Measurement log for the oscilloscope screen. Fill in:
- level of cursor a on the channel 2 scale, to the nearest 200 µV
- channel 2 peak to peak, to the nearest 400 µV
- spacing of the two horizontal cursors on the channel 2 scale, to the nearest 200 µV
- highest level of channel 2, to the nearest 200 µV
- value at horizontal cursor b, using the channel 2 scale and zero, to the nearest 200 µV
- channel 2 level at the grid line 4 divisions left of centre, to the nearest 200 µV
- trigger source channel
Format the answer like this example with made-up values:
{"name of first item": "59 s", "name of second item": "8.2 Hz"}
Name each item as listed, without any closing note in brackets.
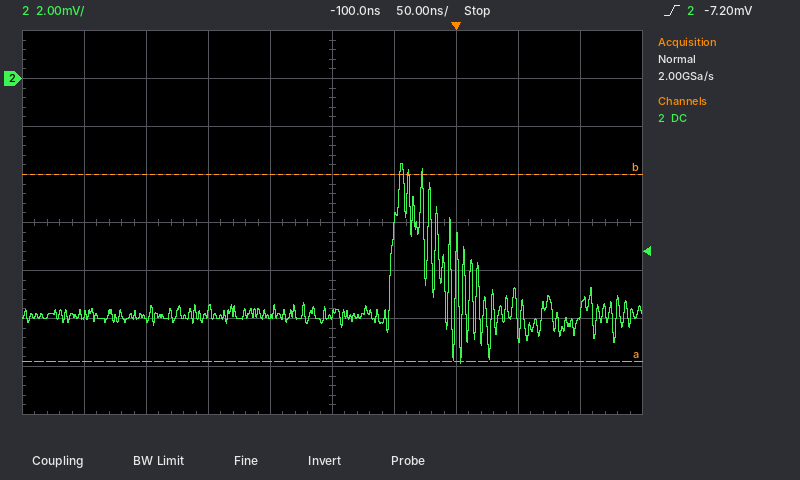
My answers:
{"level of cursor a on the channel 2 scale, to the nearest 200 µV": "-11.8 mV", "channel 2 peak to peak, to the nearest 400 µV": "8.4 mV", "spacing of the two horizontal cursors on the channel 2 scale, to the nearest 200 µV": "7.8 mV", "highest level of channel 2, to the nearest 200 µV": "-3.6 mV", "value at horizontal cursor b, using the channel 2 scale and zero, to the nearest 200 µV": "-4.0 mV", "channel 2 level at the grid line 4 divisions left of centre, to the nearest 200 µV": "-9.8 mV", "trigger source channel": "channel 2"}
